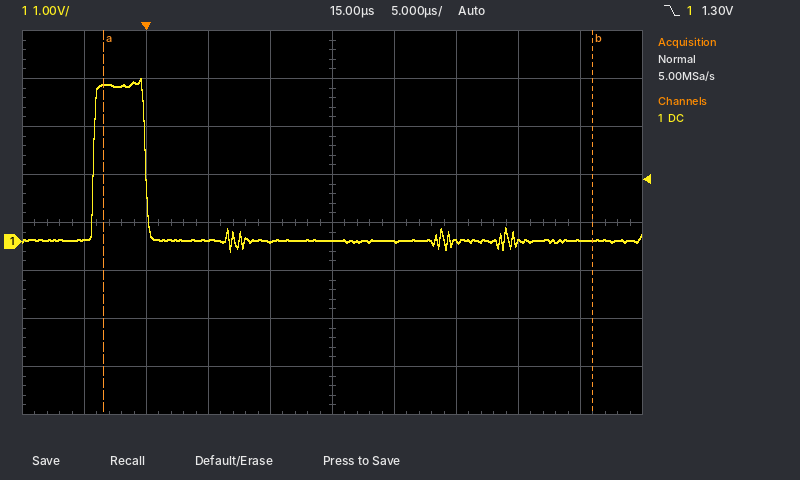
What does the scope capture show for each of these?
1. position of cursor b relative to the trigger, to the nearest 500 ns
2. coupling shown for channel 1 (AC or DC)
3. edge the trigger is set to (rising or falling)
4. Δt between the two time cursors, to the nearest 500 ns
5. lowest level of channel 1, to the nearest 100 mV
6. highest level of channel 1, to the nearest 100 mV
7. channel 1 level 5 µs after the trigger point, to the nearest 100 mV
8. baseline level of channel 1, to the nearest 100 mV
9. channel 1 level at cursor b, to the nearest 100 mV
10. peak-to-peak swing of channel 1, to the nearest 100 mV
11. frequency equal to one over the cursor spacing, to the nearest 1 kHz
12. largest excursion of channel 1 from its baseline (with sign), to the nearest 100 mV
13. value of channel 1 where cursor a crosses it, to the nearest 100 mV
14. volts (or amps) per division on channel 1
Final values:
+36.0 µs
DC
falling
39.5 µs
-200 mV
3.4 V
0.0 V
0.0 V
0.0 V
3.6 V
25 kHz
+3.4 V
3.3 V
1 V
